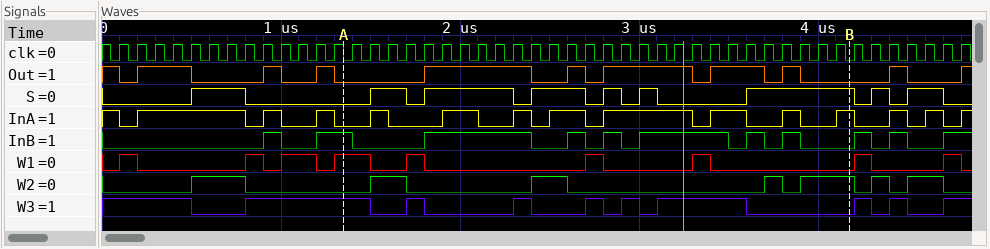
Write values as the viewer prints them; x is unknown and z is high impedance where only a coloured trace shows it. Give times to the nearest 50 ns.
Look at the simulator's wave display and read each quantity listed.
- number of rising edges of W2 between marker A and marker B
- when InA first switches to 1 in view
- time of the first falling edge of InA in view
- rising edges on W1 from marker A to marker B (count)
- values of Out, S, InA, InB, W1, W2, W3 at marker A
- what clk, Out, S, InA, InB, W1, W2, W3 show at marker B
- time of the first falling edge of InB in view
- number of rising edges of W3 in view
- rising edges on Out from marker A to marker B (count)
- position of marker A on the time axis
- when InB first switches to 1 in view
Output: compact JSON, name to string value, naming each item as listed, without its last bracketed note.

{"number of rising edges of W2 between marker A and marker B": "4", "when InA first switches to 1 in view": "200 ns", "time of the first falling edge of InA in view": "100 ns", "rising edges on W1 from marker A to marker B": "3", "values of Out, S, InA, InB, W1, W2, W3 at marker A": "Out=0, S=0, InA=0, InB=1, W1=1, W2=0, W3=1", "what clk, Out, S, InA, InB, W1, W2, W3 show at marker B": "clk=0, Out=0, S=1, InA=1, InB=0, W1=0, W2=1, W3=0", "time of the first falling edge of InB in view": "1000 ns", "number of rising edges of W3 in view": "9", "rising edges on Out from marker A to marker B": "5", "position of marker A on the time axis": "1350 ns", "when InB first switches to 1 in view": "900 ns"}
